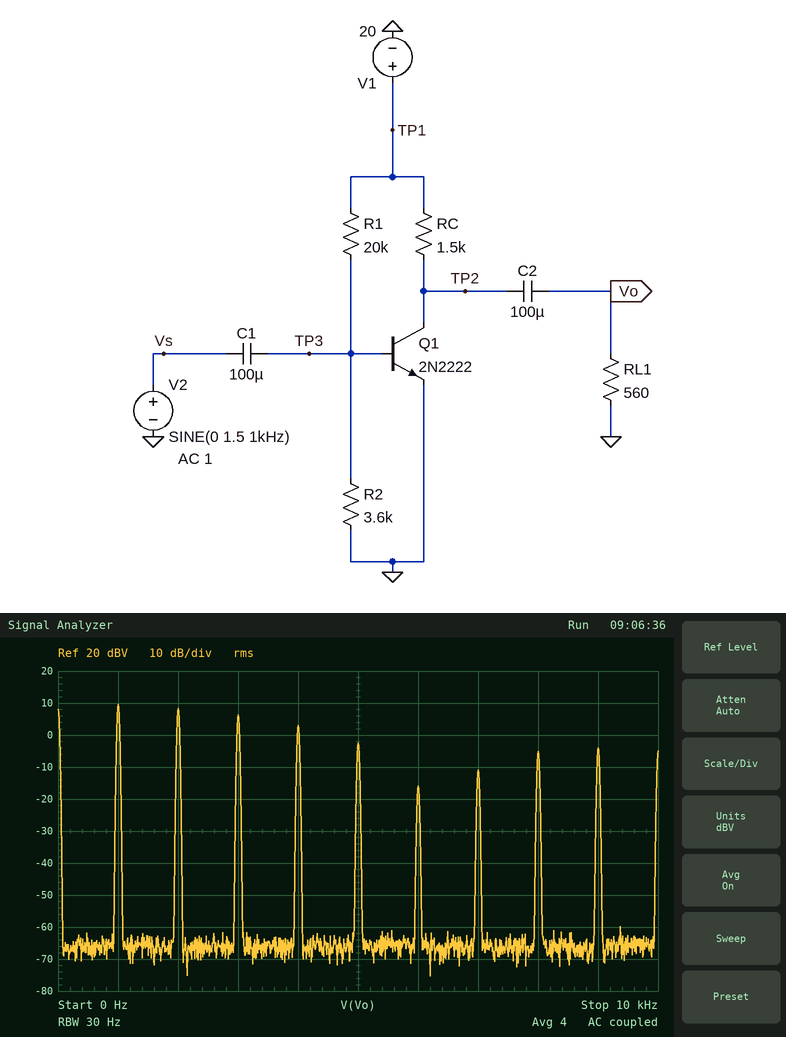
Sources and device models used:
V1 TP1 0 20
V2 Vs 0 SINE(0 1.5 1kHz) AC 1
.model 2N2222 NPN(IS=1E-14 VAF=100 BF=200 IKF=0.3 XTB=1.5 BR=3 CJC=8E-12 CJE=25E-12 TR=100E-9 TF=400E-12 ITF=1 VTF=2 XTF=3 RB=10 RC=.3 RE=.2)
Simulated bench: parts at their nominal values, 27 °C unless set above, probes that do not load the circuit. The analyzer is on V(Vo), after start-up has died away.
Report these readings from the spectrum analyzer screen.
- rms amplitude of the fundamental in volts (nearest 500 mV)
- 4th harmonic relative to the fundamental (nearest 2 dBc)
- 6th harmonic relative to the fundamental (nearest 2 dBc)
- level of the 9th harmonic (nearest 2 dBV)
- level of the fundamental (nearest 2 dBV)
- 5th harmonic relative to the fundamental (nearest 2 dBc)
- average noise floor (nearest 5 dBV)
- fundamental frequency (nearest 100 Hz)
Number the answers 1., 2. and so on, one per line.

1. 3.0 V
2. -6 dBc
3. -26 dBc
4. -4 dBV
5. 10 dBV
6. -12 dBc
7. -65 dBV
8. 1.0 kHz
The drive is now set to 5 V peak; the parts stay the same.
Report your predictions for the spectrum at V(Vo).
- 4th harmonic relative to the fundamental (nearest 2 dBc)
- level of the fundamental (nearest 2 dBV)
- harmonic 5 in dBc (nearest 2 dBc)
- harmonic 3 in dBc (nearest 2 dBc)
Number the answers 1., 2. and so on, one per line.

1. -4 dBc
2. 8 dBV
3. -6 dBc
4. -2 dBc
